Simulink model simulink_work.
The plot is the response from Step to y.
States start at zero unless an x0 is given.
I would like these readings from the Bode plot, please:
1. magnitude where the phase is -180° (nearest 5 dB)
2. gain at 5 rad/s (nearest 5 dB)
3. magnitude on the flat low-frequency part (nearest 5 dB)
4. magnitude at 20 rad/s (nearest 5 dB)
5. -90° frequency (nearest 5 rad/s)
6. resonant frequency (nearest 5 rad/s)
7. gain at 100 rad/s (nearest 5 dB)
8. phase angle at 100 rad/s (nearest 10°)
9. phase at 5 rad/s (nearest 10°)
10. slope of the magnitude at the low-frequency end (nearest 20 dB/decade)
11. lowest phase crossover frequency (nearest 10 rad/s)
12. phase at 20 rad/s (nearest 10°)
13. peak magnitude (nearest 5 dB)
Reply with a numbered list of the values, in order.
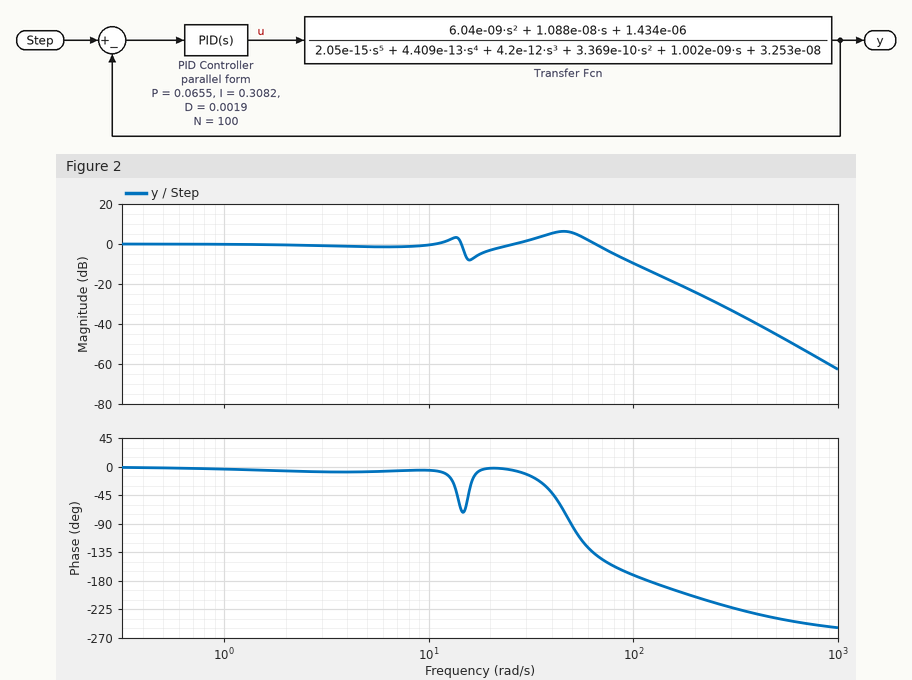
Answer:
1. -15 dB
2. 0 dB
3. 0 dB
4. -5 dB
5. 50 rad/s
6. 45 rad/s
7. -10 dB
8. -170°
9. -10°
10. 0 dB/decade
11. 120 rad/s
12. 0°
13. 5 dB
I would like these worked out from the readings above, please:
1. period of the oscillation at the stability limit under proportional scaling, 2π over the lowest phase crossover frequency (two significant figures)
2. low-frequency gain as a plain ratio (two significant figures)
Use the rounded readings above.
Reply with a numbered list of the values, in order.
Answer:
1. 0.052 s
2. 1.0
